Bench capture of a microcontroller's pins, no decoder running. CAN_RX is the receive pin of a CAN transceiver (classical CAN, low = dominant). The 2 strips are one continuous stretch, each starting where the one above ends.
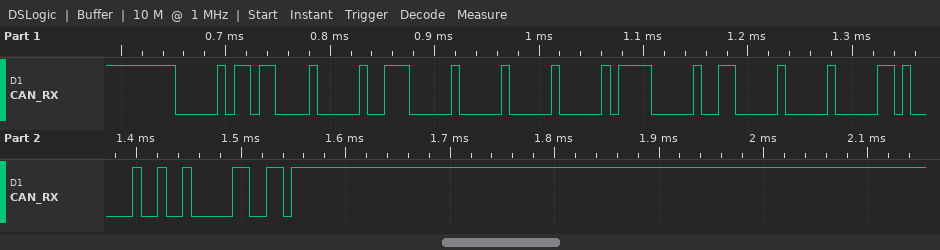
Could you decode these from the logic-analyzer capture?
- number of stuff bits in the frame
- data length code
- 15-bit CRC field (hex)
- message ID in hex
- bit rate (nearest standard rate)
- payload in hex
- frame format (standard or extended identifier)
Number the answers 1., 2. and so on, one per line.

1. 12
2. 8
3. 0x1209
4. 0x036
5. 125 kbit/s
6. 0E 00 00 0F 01 80 00 A0
7. standard
